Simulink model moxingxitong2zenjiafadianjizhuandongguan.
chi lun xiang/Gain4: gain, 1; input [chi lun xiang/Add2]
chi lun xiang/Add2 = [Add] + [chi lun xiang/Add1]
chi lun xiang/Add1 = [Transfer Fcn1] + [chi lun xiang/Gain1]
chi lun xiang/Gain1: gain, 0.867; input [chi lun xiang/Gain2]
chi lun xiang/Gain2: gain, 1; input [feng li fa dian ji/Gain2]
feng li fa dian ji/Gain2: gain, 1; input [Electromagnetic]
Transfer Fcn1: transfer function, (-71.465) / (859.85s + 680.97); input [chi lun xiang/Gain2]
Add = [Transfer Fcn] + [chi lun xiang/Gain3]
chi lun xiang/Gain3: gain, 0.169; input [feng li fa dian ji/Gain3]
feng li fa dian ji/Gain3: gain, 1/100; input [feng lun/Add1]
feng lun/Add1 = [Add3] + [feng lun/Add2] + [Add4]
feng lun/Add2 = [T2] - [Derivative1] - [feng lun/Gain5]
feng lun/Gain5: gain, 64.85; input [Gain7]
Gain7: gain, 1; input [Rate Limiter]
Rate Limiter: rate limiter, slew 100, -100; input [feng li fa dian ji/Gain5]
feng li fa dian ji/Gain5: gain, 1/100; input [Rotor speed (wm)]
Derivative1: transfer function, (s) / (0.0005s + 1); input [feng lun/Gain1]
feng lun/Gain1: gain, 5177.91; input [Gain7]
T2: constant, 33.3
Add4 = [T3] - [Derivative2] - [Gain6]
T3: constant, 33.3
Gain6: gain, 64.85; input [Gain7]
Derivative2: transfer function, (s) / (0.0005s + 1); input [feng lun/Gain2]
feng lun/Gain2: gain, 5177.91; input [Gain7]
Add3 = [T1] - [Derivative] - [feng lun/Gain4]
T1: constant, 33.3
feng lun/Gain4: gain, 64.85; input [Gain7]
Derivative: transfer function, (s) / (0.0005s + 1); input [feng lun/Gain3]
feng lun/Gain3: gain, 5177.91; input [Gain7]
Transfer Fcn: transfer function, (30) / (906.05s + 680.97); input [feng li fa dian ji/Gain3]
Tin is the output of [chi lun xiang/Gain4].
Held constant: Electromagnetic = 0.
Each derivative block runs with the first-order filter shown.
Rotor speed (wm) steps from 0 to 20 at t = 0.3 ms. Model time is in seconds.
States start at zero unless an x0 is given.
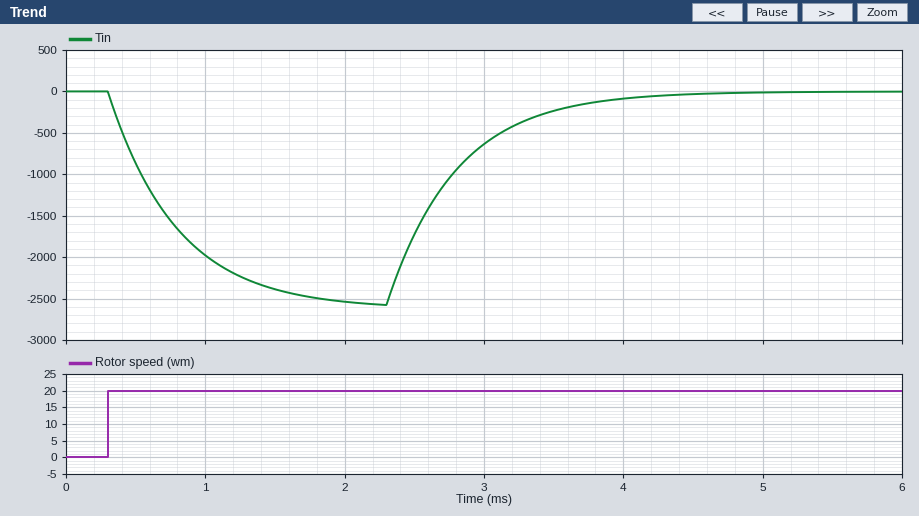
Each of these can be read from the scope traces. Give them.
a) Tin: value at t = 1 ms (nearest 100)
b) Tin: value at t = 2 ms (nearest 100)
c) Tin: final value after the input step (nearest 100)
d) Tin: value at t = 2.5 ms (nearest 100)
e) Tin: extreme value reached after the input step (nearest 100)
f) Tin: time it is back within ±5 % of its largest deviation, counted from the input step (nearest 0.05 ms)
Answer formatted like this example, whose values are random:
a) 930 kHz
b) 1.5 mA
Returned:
a) -2000
b) -2500
c) 0
d) -1700
e) -2600
f) 3.50 ms
